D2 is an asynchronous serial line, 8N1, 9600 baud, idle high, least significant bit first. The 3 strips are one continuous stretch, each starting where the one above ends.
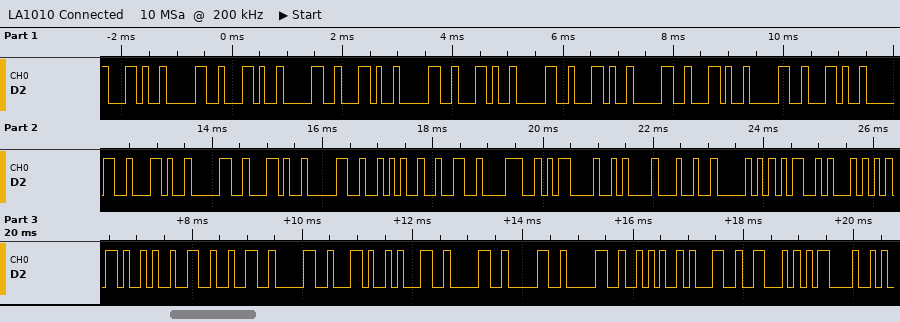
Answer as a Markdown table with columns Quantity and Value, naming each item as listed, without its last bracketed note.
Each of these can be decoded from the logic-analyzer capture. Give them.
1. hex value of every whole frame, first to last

| Quantity | Value |
|---|---|
| hex value of every whole frame, first to last | 2C 30 2C 30 2C 30 2C 30 2C 30 2C 30 2C 30 2C 30 2C 30 2A 32 38 0D 0A 24 50 4D 54 4B 32 32 30 2C 31 30 30 30 2A 31 46 0D |
